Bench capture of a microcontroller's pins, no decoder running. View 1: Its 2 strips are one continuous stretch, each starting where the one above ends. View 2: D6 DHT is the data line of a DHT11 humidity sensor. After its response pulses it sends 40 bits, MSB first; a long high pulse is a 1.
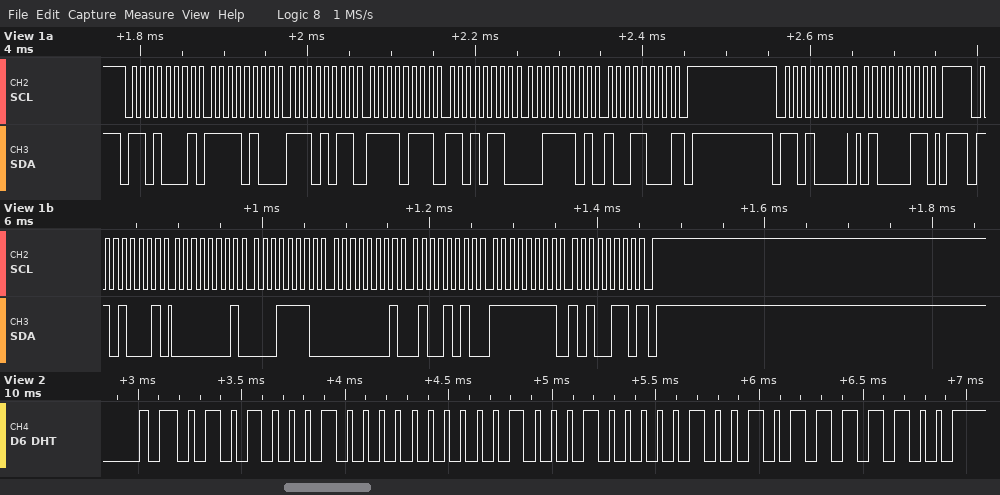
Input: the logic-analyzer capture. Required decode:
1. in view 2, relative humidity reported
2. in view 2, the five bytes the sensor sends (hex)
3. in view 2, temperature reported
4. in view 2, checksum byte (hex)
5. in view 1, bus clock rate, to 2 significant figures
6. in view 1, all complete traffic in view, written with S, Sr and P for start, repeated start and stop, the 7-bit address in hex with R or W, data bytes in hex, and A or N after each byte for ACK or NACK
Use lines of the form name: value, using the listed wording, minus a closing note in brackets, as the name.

in view 2, relative humidity reported: 81 %
in view 2, the five bytes the sensor sends: 51 00 22 09 7C
in view 2, temperature reported: 34.9 °C
in view 2, checksum byte: 0x7C
in view 1, bus clock rate, to 2 significant figures: 100 kHz
in view 1, all complete traffic in view, written with S, Sr and P for start, repeated start and stop, the 7-bit address in hex with R or W, data bytes in hex, and A or N after each byte for ACK or NACK: S 68R A F4 A EB A F7 A D6 A 3D A 98 N P S 68W A 43 A P S 68R A 01 A 1E A 01 A 4A A FF A A6 N P
